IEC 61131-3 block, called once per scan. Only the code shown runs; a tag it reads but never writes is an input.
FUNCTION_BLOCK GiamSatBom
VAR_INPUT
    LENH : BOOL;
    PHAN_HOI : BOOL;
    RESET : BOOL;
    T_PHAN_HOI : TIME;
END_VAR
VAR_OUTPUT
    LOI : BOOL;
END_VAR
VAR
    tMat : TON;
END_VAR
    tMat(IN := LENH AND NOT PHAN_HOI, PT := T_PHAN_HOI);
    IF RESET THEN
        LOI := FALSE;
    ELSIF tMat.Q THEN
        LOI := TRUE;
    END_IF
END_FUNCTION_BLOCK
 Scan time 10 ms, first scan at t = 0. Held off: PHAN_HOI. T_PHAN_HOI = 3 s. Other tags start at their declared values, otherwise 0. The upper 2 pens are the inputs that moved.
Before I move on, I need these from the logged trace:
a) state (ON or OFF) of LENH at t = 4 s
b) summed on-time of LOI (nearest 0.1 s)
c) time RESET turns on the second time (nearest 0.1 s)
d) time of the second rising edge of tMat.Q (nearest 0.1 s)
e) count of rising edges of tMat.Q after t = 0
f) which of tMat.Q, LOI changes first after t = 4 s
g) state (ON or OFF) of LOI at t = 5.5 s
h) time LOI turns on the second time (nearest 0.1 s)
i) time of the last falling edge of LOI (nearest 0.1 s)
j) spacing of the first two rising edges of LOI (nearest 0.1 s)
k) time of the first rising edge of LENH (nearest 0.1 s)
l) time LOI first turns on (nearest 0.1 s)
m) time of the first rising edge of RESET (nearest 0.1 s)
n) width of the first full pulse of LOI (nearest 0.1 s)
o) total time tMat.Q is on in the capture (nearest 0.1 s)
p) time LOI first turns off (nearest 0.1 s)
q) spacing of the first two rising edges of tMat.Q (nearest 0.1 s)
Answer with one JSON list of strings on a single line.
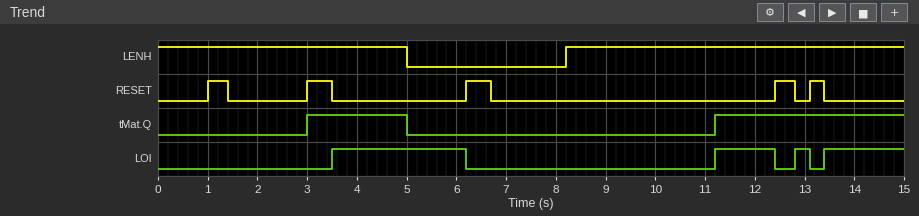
["ON", "5.8 s", "3.0 s", "11.2 s", "2", "tMat.Q", "ON", "11.2 s", "13.1 s", "7.7 s", "8.2 s", "3.5 s", "1.0 s", "2.7 s", "5.8 s", "6.2 s", "8.2 s"]
